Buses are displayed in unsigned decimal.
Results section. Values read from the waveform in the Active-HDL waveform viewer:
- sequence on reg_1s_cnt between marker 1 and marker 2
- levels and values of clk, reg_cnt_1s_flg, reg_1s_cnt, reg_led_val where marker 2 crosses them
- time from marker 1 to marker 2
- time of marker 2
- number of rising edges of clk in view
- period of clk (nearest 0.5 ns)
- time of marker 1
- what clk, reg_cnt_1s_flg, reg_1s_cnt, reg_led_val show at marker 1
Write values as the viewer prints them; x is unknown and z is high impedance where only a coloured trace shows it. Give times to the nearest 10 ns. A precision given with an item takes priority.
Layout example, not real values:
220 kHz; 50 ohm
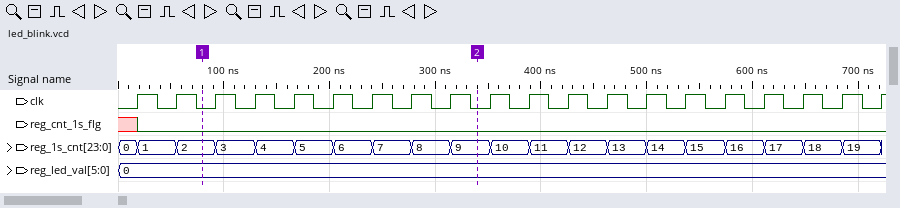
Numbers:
2, 3, 4, 5, 6, 7, 8, 9; clk=0, reg_cnt_1s_flg=0, reg_1s_cnt=9, reg_led_val=0; 260 ns; 340 ns; 20; 37 ns; 80 ns; clk=0, reg_cnt_1s_flg=0, reg_1s_cnt=2, reg_led_val=0
